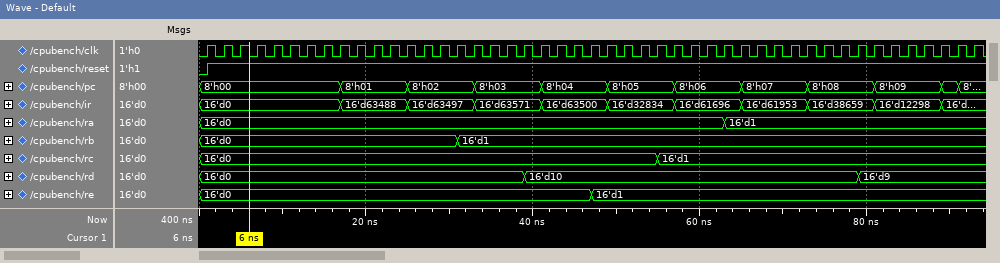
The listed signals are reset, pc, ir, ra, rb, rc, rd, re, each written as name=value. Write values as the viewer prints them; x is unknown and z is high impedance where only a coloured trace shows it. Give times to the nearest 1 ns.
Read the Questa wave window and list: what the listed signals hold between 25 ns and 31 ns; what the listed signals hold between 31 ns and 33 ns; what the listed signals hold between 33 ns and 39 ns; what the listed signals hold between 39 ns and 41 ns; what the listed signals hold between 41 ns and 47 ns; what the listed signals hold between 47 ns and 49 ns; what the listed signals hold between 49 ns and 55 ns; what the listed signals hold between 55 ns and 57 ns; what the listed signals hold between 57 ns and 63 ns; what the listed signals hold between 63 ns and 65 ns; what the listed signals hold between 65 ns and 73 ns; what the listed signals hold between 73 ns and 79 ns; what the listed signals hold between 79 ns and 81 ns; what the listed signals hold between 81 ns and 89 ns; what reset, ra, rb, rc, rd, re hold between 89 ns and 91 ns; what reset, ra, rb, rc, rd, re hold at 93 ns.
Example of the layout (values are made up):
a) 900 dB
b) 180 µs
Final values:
a) reset=1, pc=8'h02, ir=16'd63497, ra=16'd0, rb=16'd0, rc=16'd0, rd=16'd0, re=16'd0
b) reset=1, pc=8'h02, ir=16'd63497, ra=16'd0, rb=16'd1, rc=16'd0, rd=16'd0, re=16'd0
c) reset=1, pc=8'h03, ir=16'd63571, ra=16'd0, rb=16'd1, rc=16'd0, rd=16'd0, re=16'd0
d) reset=1, pc=8'h03, ir=16'd63571, ra=16'd0, rb=16'd1, rc=16'd0, rd=16'd10, re=16'd0
e) reset=1, pc=8'h04, ir=16'd63500, ra=16'd0, rb=16'd1, rc=16'd0, rd=16'd10, re=16'd0
f) reset=1, pc=8'h04, ir=16'd63500, ra=16'd0, rb=16'd1, rc=16'd0, rd=16'd10, re=16'd1
g) reset=1, pc=8'h05, ir=16'd32834, ra=16'd0, rb=16'd1, rc=16'd0, rd=16'd10, re=16'd1
h) reset=1, pc=8'h05, ir=16'd32834, ra=16'd0, rb=16'd1, rc=16'd1, rd=16'd10, re=16'd1
i) reset=1, pc=8'h06, ir=16'd61696, ra=16'd0, rb=16'd1, rc=16'd1, rd=16'd10, re=16'd1
j) reset=1, pc=8'h06, ir=16'd61696, ra=16'd1, rb=16'd1, rc=16'd1, rd=16'd10, re=16'd1
k) reset=1, pc=8'h07, ir=16'd61953, ra=16'd1, rb=16'd1, rc=16'd1, rd=16'd10, re=16'd1
l) reset=1, pc=8'h08, ir=16'd38659, ra=16'd1, rb=16'd1, rc=16'd1, rd=16'd10, re=16'd1
m) reset=1, pc=8'h08, ir=16'd38659, ra=16'd1, rb=16'd1, rc=16'd1, rd=16'd9, re=16'd1
n) reset=1, pc=8'h09, ir=16'd12298, ra=16'd1, rb=16'd1, rc=16'd1, rd=16'd9, re=16'd1
o) reset=1, ra=16'd1, rb=16'd1, rc=16'd1, rd=16'd9, re=16'd1
p) reset=1, ra=16'd1, rb=16'd1, rc=16'd1, rd=16'd9, re=16'd1
